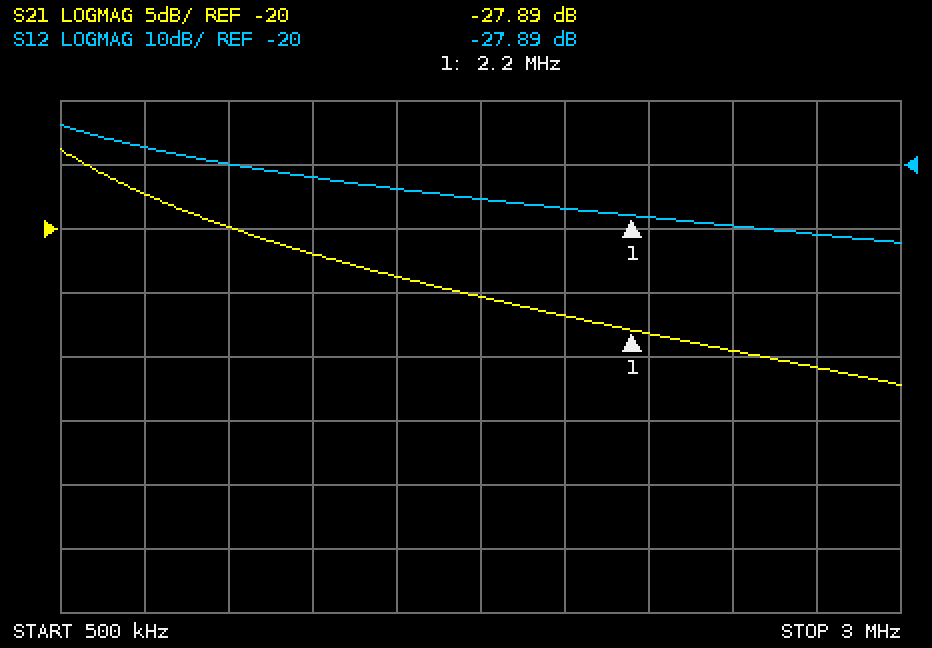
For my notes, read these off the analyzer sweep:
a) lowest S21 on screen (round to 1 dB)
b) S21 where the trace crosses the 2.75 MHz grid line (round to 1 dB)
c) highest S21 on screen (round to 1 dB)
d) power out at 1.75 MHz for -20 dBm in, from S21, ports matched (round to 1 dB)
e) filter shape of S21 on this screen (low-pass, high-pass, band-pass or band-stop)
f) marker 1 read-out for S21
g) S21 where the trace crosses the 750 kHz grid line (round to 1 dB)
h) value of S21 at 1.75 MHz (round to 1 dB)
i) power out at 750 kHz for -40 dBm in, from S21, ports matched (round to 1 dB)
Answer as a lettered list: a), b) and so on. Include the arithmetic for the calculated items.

a) -32 dB
b) -31 dB
c) -14 dB
d) -20 dBm + (-25 dB) = -45 dBm
e) low-pass
f) -27.89 dB
g) -17 dB
h) -25 dB
i) -40 dBm + (-17 dB) = -57 dBm
